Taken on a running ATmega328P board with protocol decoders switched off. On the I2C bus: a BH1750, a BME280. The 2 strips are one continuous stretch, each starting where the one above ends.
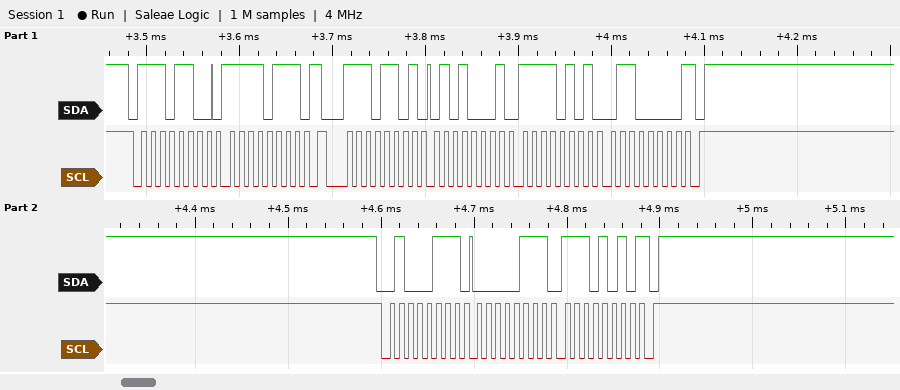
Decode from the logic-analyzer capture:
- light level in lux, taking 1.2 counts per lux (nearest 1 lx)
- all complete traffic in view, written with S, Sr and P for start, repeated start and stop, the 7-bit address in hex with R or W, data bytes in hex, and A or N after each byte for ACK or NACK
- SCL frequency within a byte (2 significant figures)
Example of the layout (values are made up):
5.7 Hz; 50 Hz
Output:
1688 lx; S 76W A F7 A Sr 76R A 51 A F5 A 60 N P S 23R A 07 A EA N P; 100 kHz
